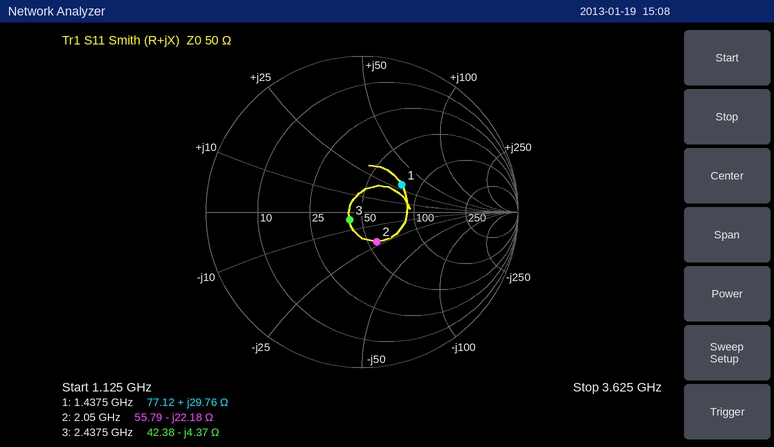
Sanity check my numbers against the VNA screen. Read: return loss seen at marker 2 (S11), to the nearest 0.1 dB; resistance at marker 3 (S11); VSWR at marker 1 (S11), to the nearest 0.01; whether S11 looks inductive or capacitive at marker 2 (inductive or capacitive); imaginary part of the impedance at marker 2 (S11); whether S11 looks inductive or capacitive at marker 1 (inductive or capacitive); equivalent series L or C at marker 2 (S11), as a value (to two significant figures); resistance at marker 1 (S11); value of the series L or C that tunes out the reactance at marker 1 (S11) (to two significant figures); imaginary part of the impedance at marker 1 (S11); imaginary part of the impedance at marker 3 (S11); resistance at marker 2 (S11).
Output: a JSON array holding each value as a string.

["13.5 dB", "42.38 Ω", "1.89", "capacitive", "-22.18 Ω", "inductive", "3.5 pF", "77.12 Ω", "3.7 pF", "+29.76 Ω", "-4.37 Ω", "55.79 Ω"]
